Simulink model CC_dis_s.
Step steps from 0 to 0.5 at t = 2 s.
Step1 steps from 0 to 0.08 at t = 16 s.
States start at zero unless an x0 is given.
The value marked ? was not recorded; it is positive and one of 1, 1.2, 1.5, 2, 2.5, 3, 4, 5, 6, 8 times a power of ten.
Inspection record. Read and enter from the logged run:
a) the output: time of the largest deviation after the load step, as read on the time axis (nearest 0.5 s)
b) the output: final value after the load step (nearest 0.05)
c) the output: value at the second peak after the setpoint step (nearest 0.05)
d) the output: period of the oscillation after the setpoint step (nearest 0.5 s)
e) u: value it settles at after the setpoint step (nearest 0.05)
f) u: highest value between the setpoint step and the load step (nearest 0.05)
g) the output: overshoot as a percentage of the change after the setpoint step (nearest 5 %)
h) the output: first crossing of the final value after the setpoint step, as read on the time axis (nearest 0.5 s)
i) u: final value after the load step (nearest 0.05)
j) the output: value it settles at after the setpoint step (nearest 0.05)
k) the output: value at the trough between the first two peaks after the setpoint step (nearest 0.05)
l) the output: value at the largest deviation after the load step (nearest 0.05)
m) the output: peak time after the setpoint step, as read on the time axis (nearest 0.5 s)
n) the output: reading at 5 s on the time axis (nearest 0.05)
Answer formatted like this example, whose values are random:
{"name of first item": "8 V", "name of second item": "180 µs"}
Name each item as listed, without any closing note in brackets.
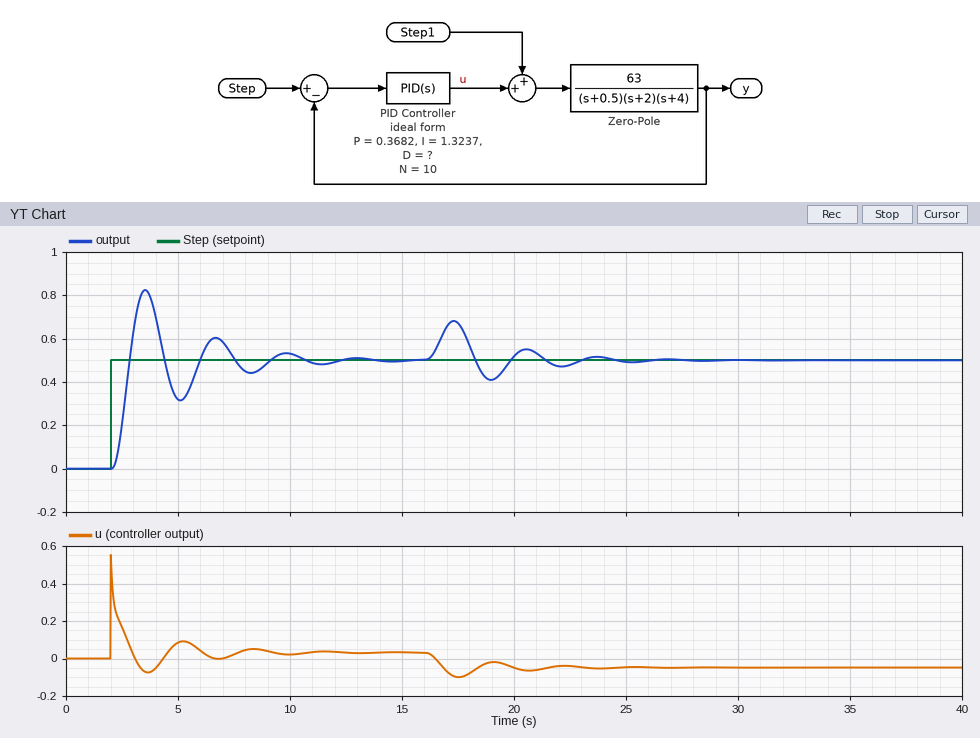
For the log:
{"the output: time of the largest deviation after the load step, as read on the time axis": "17.5 s", "the output: final value after the load step": "0.50", "the output: value at the second peak after the setpoint step": "0.60", "the output: period of the oscillation after the setpoint step": "3.0 s", "u: value it settles at after the setpoint step": "0.05", "u: highest value between the setpoint step and the load step": "0.55", "the output: overshoot as a percentage of the change after the setpoint step": "65 %", "the output: first crossing of the final value after the setpoint step, as read on the time axis": "3.0 s", "u: final value after the load step": "-0.05", "the output: value it settles at after the setpoint step": "0.50", "the output: value at the trough between the first two peaks after the setpoint step": "0.30", "the output: value at the largest deviation after the load step": "0.70", "the output: peak time after the setpoint step, as read on the time axis": "3.5 s", "the output: reading at 5 s on the time axis": "0.30"}
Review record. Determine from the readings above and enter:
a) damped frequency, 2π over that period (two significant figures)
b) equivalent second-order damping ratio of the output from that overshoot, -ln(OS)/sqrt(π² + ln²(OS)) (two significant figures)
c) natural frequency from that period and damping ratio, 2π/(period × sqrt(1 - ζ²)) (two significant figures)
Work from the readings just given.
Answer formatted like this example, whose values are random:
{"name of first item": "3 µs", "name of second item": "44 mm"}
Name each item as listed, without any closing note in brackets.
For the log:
{"damped frequency, 2π over that period": "2.1 rad/s", "equivalent second-order damping ratio of the output from that overshoot, -ln(OS)/sqrt(π² + ln²(OS))": "0.14", "natural frequency from that period and damping ratio, 2π/(period × sqrt(1 - ζ²))": "2.1 rad/s"}
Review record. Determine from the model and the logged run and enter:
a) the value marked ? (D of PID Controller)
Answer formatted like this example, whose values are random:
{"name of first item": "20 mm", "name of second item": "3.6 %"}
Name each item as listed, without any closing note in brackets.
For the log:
{"the value marked ?": "0.2"}
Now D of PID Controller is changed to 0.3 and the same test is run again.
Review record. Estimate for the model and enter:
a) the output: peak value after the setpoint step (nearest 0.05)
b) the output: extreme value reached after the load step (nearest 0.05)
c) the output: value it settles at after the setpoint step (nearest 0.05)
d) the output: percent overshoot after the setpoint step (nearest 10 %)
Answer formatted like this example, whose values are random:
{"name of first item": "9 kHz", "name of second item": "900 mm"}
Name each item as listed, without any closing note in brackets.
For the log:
{"the output: peak value after the setpoint step": "0.75", "the output: extreme value reached after the load step": "0.65", "the output: value it settles at after the setpoint step": "0.50", "the output: percent overshoot after the setpoint step": "50 %"}
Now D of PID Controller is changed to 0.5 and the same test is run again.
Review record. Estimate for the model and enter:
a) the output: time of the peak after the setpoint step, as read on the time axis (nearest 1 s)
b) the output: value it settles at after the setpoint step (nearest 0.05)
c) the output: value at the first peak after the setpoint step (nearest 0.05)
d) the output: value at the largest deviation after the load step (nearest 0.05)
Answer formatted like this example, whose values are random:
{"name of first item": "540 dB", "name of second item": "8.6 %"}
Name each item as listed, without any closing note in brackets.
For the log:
{"the output: time of the peak after the setpoint step, as read on the time axis": "3 s", "the output: value it settles at after the setpoint step": "0.50", "the output: value at the first peak after the setpoint step": "0.65", "the output: value at the largest deviation after the load step": "0.65"}
